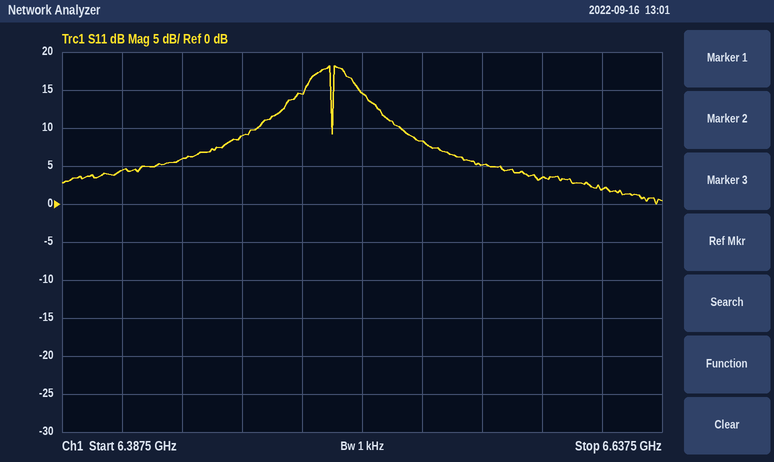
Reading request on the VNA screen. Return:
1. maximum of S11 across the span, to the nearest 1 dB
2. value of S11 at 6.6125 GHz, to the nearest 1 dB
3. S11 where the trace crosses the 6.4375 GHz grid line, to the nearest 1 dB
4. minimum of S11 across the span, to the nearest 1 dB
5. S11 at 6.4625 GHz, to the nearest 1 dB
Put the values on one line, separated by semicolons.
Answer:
18 dB; 2 dB; 6 dB; 0 dB; 9 dB
